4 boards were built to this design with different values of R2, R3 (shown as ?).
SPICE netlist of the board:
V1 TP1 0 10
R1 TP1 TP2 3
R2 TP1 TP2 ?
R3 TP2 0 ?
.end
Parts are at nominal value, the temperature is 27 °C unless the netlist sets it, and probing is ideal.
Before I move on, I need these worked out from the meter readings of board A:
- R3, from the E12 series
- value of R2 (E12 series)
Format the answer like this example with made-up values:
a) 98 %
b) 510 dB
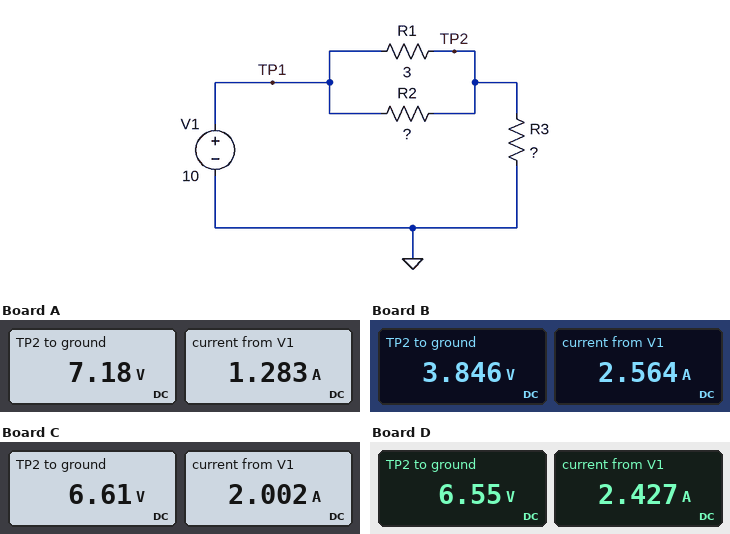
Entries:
a) 5.6 Ω
b) 8.2 Ω
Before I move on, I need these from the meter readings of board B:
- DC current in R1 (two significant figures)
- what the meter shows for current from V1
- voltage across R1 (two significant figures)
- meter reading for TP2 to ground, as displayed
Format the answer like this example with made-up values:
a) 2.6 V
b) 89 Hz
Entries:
a) 2.1 A
b) 2.564 A
c) 6.2 V
d) 3.846 V
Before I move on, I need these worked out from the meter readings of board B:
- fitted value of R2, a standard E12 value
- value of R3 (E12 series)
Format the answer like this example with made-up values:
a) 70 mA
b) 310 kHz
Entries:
a) 12 Ω
b) 1.5 Ω
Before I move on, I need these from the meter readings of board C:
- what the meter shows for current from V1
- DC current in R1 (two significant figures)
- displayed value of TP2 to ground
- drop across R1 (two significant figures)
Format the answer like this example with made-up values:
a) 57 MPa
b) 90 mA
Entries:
a) 2.002 A
b) 1.1 A
c) 6.61 V
d) 3.4 V
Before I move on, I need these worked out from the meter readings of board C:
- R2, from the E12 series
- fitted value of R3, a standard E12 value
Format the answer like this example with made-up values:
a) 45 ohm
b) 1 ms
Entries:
a) 3.9 Ω
b) 3.3 Ω
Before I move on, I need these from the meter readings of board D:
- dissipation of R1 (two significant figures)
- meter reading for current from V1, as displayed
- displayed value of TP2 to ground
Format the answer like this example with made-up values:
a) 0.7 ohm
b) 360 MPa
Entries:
a) 4.0 W
b) 2.427 A
c) 6.55 V
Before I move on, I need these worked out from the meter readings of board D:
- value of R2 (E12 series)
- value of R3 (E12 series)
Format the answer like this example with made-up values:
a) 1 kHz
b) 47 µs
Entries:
a) 2.7 Ω
b) 2.7 Ω
